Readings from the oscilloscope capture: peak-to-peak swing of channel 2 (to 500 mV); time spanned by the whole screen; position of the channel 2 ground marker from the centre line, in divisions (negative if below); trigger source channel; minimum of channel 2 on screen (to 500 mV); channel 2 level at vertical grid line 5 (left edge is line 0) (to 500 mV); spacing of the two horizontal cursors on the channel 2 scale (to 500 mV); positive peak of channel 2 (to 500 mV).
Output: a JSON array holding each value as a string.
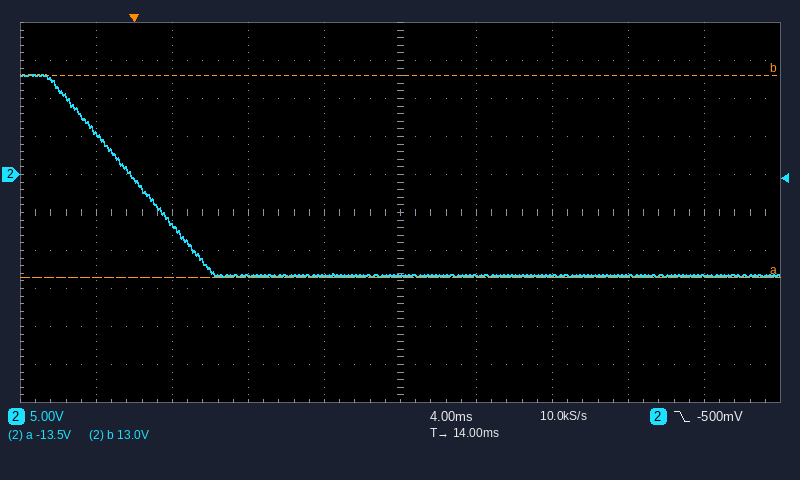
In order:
["26.5 V", "40 ms", "+1.0 div", "channel 2", "-13.5 V", "-13.5 V", "26.5 V", "13.0 V"]
